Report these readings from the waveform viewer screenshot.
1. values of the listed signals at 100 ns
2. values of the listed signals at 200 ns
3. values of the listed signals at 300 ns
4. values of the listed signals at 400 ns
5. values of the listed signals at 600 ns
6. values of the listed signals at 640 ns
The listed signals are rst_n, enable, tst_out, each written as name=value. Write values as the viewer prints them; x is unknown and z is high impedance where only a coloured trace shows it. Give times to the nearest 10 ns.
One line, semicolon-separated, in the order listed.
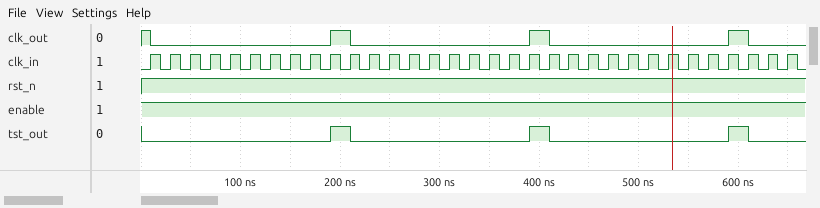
rst_n=1, enable=1, tst_out=0; rst_n=1, enable=1, tst_out=1; rst_n=1, enable=1, tst_out=0; rst_n=1, enable=1, tst_out=1; rst_n=1, enable=1, tst_out=1; rst_n=1, enable=1, tst_out=0
